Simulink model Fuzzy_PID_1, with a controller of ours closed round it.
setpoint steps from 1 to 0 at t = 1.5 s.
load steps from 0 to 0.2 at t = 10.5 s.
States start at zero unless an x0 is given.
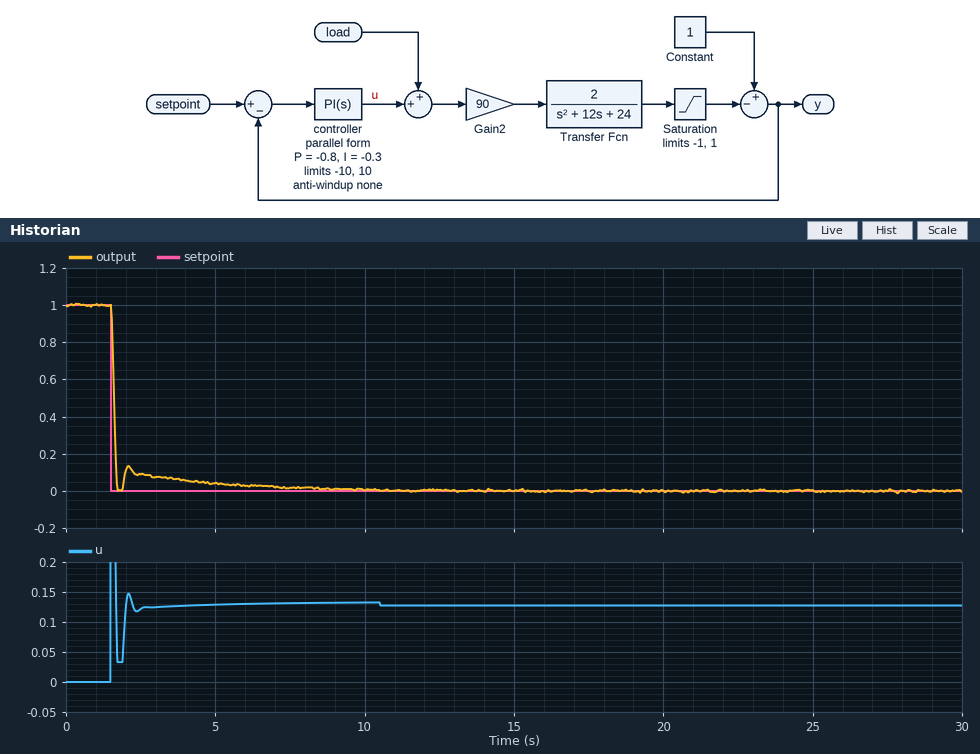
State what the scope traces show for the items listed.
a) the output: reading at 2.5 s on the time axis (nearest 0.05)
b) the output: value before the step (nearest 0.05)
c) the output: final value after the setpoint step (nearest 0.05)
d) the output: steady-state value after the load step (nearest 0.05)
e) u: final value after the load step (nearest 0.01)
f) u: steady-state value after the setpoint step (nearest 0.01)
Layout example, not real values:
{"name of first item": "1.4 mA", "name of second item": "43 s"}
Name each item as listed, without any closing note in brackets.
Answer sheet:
{"the output: reading at 2.5 s on the time axis": "0.10", "the output: value before the step": "1.00", "the output: final value after the setpoint step": "0.00", "the output: steady-state value after the load step": "0.00", "u: final value after the load step": "0.13", "u: steady-state value after the setpoint step": "0.13"}
